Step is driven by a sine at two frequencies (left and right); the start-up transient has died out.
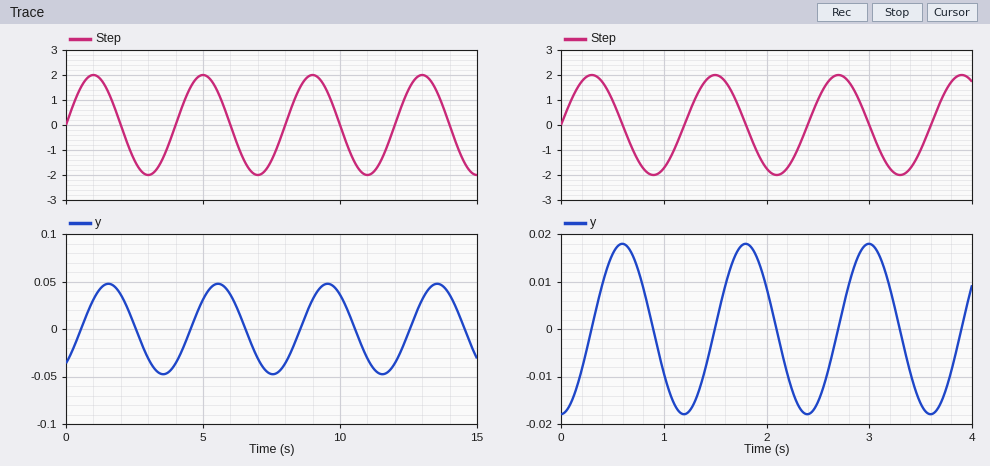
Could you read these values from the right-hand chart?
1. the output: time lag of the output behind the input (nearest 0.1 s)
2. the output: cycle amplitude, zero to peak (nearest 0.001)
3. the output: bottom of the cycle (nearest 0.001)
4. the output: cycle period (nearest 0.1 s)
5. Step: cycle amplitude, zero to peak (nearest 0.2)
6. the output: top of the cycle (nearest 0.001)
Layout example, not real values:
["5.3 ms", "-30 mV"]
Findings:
["0.3 s", "0.018", "-0.018", "1.2 s", "2.0", "0.018"]
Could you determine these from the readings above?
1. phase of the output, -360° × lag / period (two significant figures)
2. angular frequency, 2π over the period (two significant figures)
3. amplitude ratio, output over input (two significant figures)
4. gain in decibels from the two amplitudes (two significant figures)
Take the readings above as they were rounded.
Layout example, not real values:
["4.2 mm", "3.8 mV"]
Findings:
["-90°", "5.2 rad/s", "0.0090", "-41 dB"]
